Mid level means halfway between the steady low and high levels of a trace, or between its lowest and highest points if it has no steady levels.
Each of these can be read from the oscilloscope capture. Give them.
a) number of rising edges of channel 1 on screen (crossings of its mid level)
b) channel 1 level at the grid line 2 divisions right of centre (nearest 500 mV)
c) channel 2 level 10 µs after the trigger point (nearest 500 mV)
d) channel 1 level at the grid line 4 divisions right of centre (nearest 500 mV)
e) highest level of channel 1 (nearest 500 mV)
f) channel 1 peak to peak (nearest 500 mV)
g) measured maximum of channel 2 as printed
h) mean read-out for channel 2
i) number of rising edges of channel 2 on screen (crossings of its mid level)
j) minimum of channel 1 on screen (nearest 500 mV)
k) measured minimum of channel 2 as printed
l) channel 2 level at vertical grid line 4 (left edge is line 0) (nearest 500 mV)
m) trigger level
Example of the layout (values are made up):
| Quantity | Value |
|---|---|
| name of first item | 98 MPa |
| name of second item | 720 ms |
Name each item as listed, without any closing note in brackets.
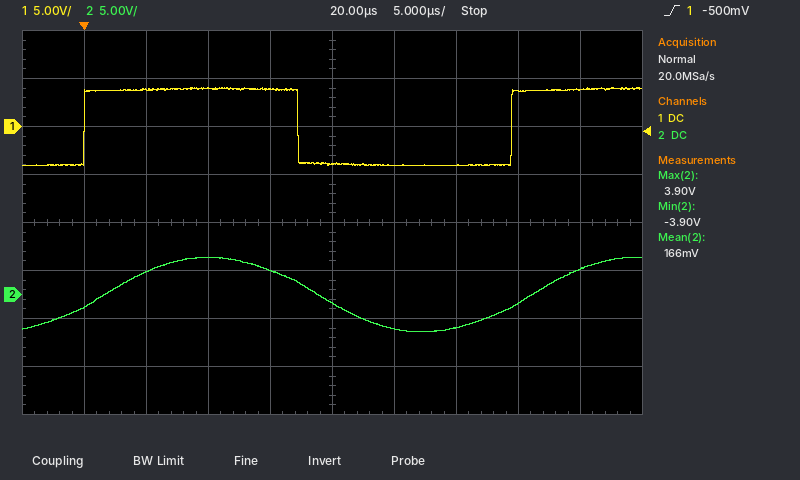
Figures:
| Quantity | Value |
|---|---|
| number of rising edges of channel 1 on screen | 2 |
| channel 1 level at the grid line 2 divisions right of centre | -4.0 V |
| channel 2 level 10 µs after the trigger point | 4.0 V |
| channel 1 level at the grid line 4 divisions right of centre | 4.0 V |
| highest level of channel 1 | 4.0 V |
| channel 1 peak to peak | 8.0 V |
| measured maximum of channel 2 as printed | 3.90 V |
| mean read-out for channel 2 | 166 mV |
| number of rising edges of channel 2 on screen | 2 |
| minimum of channel 1 on screen | -4.0 V |
| measured minimum of channel 2 as printed | -3.90 V |
| channel 2 level at vertical grid line 4 (left edge is line 0) | 2.5 V |
| trigger level | -500 mV |
